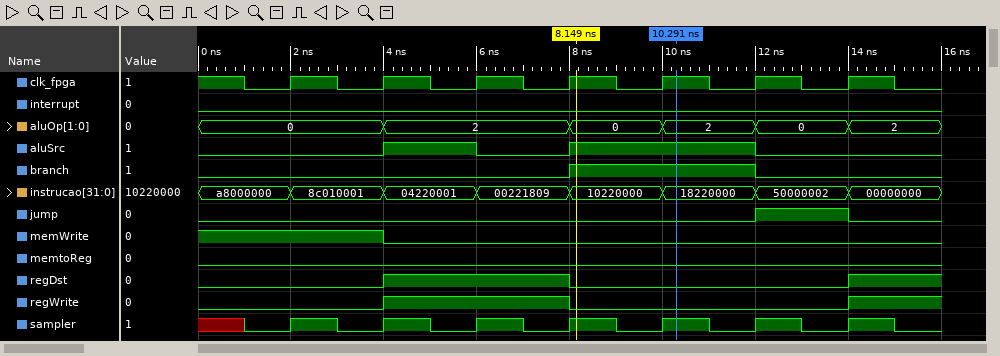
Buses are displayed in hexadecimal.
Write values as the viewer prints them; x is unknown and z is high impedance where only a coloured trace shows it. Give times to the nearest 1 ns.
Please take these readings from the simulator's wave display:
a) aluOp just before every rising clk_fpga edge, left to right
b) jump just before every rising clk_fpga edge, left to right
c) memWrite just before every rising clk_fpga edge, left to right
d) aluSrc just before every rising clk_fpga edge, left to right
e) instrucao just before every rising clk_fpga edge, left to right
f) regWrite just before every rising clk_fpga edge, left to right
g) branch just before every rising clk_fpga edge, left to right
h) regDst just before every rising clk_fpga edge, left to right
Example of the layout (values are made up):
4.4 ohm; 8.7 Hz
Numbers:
0, 0, 2, 2, 0, 2, 0; 0 0 0 0 0 0 1; 1 1 0 0 0 0 0; 0 0 1 0 1 1 0; a8000000, 8c010001, 04220001, 00221809, 10220000, 18220000, 50000002; 0 0 1 1 0 0 0; 0 0 0 0 1 1 0; 0 0 1 1 0 0 0
